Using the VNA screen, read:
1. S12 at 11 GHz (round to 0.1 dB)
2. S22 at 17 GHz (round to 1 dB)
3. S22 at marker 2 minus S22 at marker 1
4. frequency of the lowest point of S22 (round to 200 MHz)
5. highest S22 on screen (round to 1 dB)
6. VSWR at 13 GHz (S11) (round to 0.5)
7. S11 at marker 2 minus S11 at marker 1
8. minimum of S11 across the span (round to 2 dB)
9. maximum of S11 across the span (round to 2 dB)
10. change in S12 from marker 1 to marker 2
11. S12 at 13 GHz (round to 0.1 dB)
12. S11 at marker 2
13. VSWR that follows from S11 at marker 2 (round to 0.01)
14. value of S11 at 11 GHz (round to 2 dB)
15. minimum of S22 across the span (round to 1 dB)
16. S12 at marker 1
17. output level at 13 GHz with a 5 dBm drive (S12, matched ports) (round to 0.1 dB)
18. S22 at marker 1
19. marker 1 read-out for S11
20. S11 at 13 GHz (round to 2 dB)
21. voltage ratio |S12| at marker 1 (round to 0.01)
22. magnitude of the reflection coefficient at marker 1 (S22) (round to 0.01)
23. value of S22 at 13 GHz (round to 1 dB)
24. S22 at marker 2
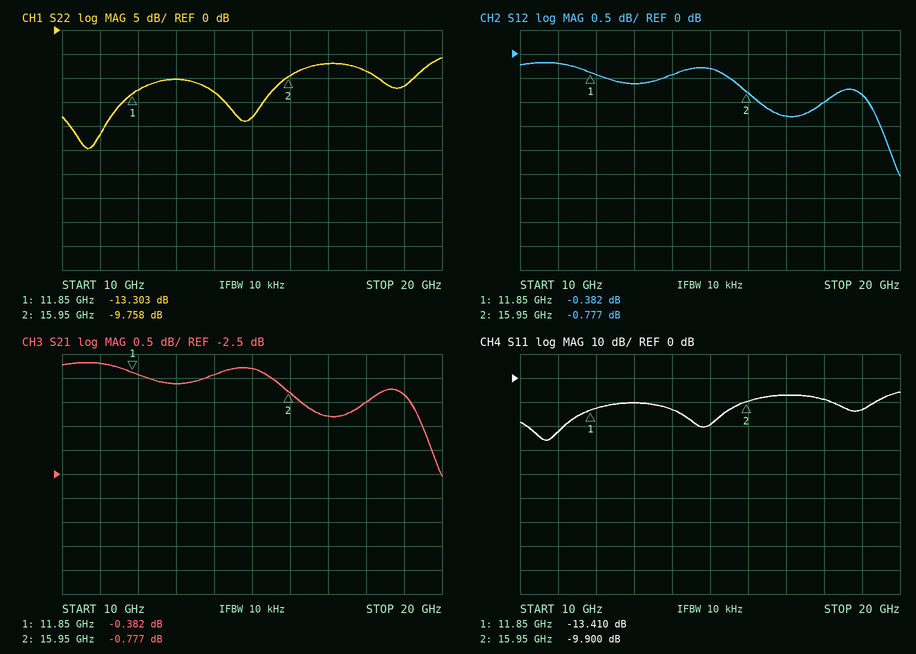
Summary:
-0.2 dB
-7 dB
3.545 dB
10.6 GHz
-6 dB
2.0
3.510 dB
-26 dB
-6 dB
-0.395 dB
-0.6 dB
-9.900 dB
1.94
-22 dB
-25 dB
-0.382 dB
4.4 dBm
-13.303 dB
-13.410 dB
-10 dB
0.96
0.22
-10 dB
-9.758 dB
